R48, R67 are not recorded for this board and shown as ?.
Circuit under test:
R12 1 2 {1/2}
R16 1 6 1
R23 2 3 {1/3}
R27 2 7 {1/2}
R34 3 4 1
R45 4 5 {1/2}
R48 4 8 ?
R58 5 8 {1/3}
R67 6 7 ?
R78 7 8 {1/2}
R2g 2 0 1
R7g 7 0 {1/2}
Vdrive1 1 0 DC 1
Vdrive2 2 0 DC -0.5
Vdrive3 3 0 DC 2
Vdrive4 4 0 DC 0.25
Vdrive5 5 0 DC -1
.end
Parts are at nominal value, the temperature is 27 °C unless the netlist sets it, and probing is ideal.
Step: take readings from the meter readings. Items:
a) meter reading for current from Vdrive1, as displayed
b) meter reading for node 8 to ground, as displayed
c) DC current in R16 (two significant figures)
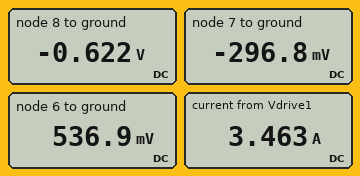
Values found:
3.463 A
-0.622 V
460 mA
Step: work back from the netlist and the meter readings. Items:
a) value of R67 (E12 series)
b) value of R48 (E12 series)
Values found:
1.8 Ω
1.8 Ω
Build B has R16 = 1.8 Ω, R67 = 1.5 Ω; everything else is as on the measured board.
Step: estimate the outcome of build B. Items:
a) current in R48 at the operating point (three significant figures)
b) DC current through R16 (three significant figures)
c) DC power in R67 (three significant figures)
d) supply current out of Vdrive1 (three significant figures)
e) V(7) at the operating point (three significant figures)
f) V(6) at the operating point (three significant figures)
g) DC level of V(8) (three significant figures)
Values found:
487 mA
397 mA
236 mW
3.40 A
-309 mV
286 mV
-626 mV
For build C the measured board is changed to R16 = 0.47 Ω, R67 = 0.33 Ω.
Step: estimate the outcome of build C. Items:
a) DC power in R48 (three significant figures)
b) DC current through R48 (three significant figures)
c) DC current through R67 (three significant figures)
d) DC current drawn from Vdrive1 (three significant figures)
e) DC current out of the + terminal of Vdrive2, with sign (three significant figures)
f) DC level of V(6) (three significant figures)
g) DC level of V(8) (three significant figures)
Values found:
363 mW
449 mA
1.40 A
4.40 A
-11.8 A
342 mV
-558 mV
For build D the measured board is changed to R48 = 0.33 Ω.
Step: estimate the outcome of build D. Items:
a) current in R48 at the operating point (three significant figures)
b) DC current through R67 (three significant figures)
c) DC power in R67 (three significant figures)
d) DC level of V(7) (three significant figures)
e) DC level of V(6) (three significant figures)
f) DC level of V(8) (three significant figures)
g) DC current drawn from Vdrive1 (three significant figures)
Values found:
1.76 A
430 mA
333 mW
-205 mV
570 mV
-330 mV
3.43 A
